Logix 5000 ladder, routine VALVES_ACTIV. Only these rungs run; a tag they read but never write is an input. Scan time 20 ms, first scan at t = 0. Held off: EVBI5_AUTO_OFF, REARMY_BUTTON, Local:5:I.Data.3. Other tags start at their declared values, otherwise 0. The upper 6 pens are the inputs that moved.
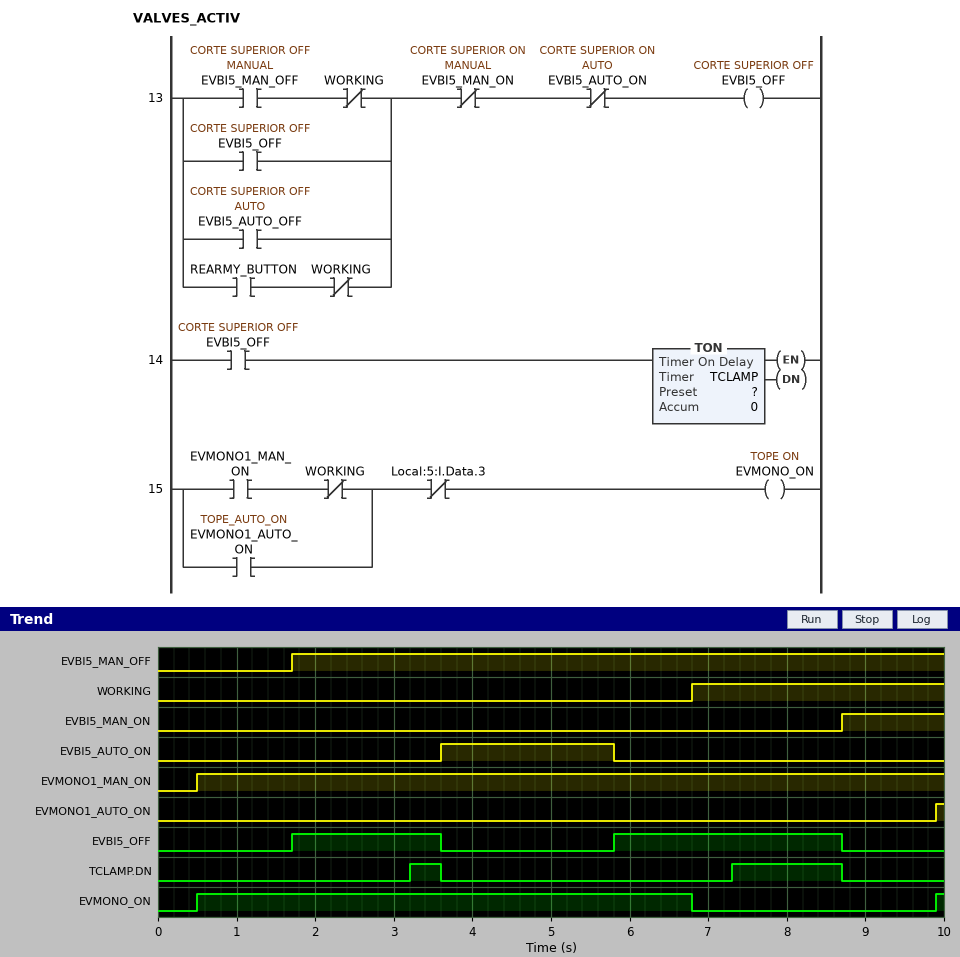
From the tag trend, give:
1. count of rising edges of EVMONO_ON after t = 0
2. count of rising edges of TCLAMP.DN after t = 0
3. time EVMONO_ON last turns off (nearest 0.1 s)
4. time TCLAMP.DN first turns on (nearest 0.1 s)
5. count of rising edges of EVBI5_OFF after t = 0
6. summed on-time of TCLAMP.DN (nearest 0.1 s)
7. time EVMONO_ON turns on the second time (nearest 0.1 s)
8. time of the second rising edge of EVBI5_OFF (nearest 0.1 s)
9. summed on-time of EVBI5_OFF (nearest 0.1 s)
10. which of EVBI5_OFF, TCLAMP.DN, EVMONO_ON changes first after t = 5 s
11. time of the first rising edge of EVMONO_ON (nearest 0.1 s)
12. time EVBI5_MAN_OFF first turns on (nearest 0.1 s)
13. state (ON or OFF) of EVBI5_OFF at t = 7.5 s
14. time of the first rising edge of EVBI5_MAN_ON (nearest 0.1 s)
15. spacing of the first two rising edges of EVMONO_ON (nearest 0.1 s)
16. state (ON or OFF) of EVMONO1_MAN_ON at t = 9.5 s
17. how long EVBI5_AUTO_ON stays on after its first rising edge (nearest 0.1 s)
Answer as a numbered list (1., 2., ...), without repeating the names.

1. 2
2. 2
3. 6.8 s
4. 3.2 s
5. 2
6. 1.8 s
7. 9.9 s
8. 5.8 s
9. 4.8 s
10. EVBI5_OFF
11. 0.5 s
12. 1.7 s
13. ON
14. 8.7 s
15. 9.4 s
16. ON
17. 2.2 s
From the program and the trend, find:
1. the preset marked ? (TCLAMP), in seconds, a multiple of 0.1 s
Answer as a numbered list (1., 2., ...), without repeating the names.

1. 1.5 s
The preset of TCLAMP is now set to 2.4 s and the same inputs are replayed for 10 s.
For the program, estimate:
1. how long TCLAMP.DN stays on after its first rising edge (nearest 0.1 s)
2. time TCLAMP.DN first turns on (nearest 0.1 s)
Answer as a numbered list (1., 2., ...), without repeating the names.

1. 0.5 s
2. 8.2 s
